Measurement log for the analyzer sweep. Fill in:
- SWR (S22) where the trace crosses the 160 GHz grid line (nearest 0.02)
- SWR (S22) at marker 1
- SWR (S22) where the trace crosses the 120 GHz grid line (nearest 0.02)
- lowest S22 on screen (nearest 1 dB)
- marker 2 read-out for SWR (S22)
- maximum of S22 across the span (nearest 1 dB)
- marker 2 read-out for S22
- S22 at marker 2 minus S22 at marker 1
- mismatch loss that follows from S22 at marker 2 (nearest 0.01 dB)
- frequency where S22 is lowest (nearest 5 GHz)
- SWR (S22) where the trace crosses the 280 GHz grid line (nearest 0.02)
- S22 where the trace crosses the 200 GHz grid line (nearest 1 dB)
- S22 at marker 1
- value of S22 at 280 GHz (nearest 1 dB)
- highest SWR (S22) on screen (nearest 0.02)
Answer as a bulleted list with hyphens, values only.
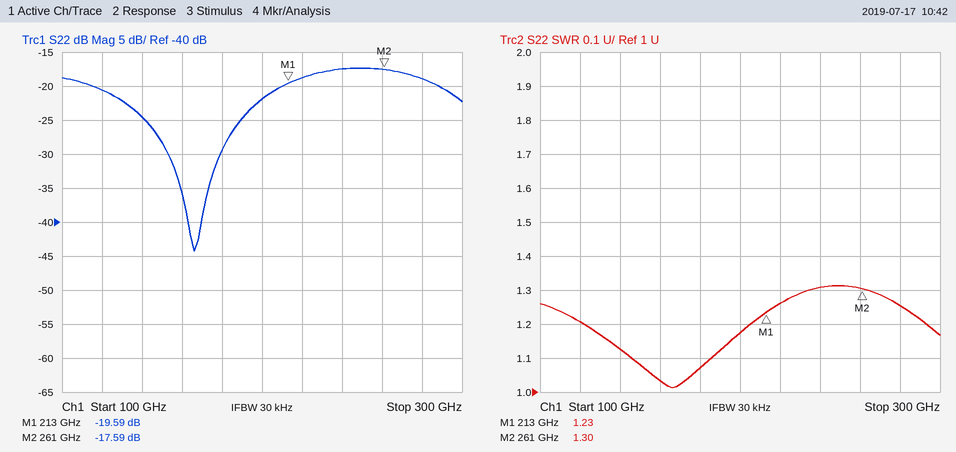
- 1.04
- 1.23
- 1.20
- -44 dB
- 1.30
- -17 dB
- -17.59 dB
- 2.00 dB
- 0.08 dB
- 165 GHz
- 1.26
- -22 dB
- -19.59 dB
- -19 dB
- 1.32
